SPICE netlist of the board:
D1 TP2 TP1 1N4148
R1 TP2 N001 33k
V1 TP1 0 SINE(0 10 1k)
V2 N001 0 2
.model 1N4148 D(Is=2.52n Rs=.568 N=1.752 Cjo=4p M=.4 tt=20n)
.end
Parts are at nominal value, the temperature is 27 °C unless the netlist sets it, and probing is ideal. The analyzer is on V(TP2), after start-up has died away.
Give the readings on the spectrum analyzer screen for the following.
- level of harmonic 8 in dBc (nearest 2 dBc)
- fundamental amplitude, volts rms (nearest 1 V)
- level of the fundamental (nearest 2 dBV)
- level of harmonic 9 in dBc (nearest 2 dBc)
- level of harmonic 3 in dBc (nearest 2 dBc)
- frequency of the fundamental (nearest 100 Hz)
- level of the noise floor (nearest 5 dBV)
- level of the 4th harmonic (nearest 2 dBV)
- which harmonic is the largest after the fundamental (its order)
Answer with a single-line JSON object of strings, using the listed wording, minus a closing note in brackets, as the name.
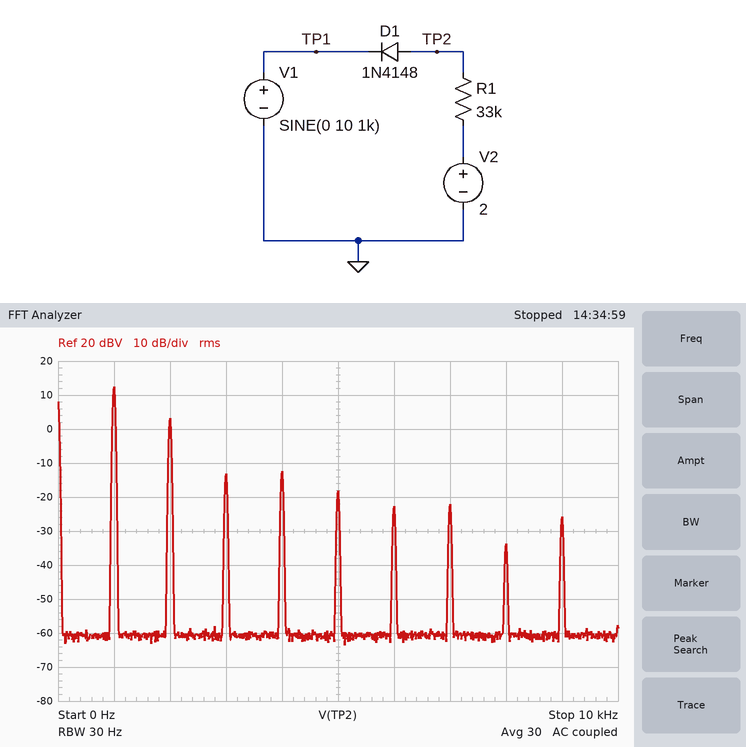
{"level of harmonic 8 in dBc": "-46 dBc", "fundamental amplitude, volts rms": "4 V", "level of the fundamental": "12 dBV", "level of harmonic 9 in dBc": "-38 dBc", "level of harmonic 3 in dBc": "-26 dBc", "frequency of the fundamental": "1.0 kHz", "level of the noise floor": "-60 dBV", "level of the 4th harmonic": "-12 dBV", "which harmonic is the largest after the fundamental": "2"}
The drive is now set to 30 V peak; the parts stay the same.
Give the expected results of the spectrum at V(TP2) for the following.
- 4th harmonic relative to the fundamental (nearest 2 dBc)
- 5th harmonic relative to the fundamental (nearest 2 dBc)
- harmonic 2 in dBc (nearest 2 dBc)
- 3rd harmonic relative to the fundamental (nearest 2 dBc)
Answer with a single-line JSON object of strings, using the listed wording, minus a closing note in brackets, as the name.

{"4th harmonic relative to the fundamental": "-22 dBc", "5th harmonic relative to the fundamental": "-38 dBc", "harmonic 2 in dBc": "-8 dBc", "3rd harmonic relative to the fundamental": "-34 dBc"}
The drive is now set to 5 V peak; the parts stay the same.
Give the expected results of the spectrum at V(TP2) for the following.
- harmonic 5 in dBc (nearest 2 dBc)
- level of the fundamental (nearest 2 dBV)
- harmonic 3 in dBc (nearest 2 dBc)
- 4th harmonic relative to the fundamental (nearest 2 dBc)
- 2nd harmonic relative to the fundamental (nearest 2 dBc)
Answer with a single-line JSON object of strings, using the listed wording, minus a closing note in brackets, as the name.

{"harmonic 5 in dBc": "-30 dBc", "level of the fundamental": "8 dBV", "harmonic 3 in dBc": "-22 dBc", "4th harmonic relative to the fundamental": "-34 dBc", "2nd harmonic relative to the fundamental": "-12 dBc"}
